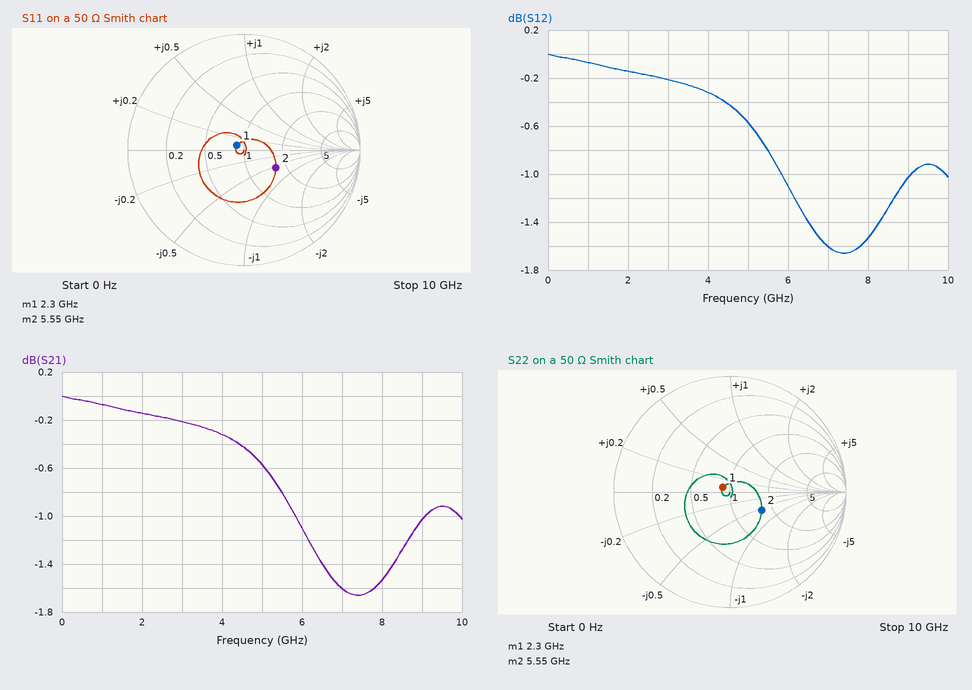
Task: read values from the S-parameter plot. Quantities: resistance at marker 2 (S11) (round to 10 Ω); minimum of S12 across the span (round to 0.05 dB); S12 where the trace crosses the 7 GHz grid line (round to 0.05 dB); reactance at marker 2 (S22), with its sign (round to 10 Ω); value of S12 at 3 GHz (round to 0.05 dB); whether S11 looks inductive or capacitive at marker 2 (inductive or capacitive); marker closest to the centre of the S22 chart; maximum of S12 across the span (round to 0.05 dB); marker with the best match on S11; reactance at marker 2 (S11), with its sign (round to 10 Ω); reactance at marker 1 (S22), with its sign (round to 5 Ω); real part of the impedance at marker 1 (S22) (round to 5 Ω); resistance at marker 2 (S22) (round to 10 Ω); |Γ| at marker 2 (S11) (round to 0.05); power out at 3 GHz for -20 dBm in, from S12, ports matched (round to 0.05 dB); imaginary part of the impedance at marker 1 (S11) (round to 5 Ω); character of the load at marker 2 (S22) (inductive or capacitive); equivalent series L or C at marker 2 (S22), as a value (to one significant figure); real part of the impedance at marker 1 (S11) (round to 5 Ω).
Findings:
80 Ω
-1.65 dB
-1.60 dB
-30 Ω
-0.20 dB
capacitive
marker 1
0.00 dB
marker 1
-30 Ω
+5 Ω
45 Ω
80 Ω
0.30
-20.20 dBm
+5 Ω
capacitive
1 pF
45 Ω
